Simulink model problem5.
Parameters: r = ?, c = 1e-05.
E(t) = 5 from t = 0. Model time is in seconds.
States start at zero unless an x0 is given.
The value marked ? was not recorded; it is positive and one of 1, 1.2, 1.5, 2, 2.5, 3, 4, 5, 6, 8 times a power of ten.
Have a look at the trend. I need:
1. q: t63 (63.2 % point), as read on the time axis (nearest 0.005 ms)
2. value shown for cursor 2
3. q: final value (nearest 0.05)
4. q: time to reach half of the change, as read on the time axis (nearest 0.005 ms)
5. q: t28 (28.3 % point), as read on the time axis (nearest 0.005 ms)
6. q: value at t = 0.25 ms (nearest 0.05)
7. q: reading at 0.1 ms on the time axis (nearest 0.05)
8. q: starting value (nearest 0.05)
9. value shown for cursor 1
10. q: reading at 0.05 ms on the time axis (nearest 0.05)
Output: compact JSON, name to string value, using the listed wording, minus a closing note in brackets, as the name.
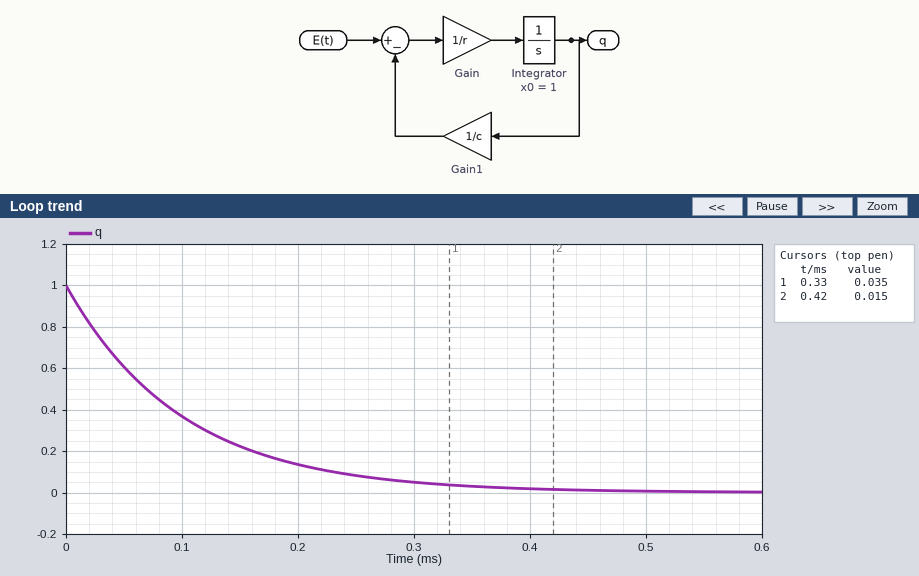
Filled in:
{"q: t63 (63.2 % point), as read on the time axis": "0.100 ms", "value shown for cursor 2": "0.015", "q: final value": "0.00", "q: time to reach half of the change, as read on the time axis": "0.070 ms", "q: t28 (28.3 % point), as read on the time axis": "0.035 ms", "q: value at t = 0.25 ms": "0.10", "q: reading at 0.1 ms on the time axis": "0.35", "q: starting value": "1.00", "value shown for cursor 1": "0.035", "q: reading at 0.05 ms on the time axis": "0.60"}
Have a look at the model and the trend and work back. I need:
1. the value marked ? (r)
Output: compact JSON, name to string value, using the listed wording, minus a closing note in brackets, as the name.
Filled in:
{"the value marked ?": "10"}
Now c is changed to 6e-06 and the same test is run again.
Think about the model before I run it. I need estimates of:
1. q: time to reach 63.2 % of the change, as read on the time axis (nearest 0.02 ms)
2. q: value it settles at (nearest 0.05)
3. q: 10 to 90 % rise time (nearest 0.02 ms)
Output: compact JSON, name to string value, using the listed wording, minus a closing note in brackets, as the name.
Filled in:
{"q: time to reach 63.2 % of the change, as read on the time axis": "0.06 ms", "q: value it settles at": "0.00", "q: 10 to 90 % rise time": "0.14 ms"}
